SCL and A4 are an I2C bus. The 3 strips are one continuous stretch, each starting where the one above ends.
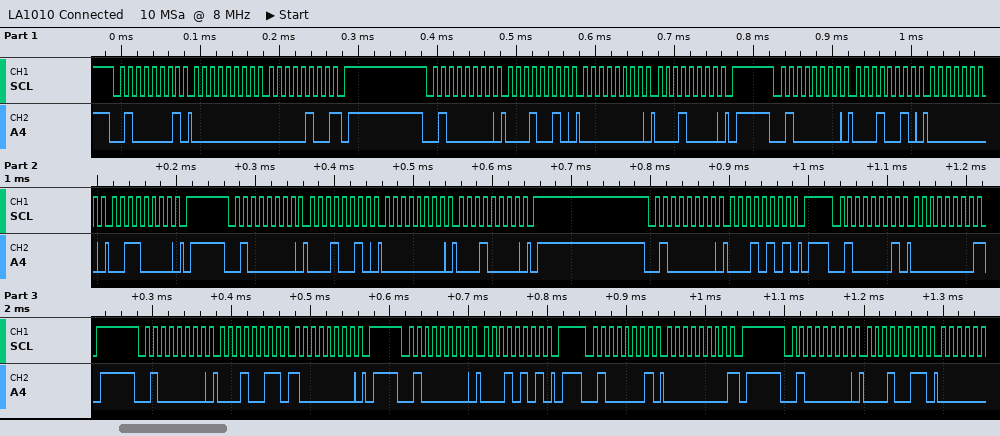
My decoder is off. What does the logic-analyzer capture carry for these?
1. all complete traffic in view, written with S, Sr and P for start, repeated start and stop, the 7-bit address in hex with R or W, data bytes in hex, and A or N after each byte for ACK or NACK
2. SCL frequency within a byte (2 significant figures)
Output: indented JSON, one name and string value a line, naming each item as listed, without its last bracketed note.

{
  "all complete traffic in view, written with S, Sr and P for start, repeated start and stop, the 7-bit address in hex with R or W, data bytes in hex, and A or N after each byte for ACK or NACK": "S 20R A 00 A 04 N P S 20W A 12 A 00 A 10 A P S 20W A 12 A 00 A 30 A P S 20W A 12 A 00 A 10 A P S 20W A 15 A P S 20R A 00 N P S 20W A 13 A 80 A P S 20W A 15 A P S 20R A 00 N P S 20W A 13 A",
  "SCL frequency within a byte": "100 kHz"
}
